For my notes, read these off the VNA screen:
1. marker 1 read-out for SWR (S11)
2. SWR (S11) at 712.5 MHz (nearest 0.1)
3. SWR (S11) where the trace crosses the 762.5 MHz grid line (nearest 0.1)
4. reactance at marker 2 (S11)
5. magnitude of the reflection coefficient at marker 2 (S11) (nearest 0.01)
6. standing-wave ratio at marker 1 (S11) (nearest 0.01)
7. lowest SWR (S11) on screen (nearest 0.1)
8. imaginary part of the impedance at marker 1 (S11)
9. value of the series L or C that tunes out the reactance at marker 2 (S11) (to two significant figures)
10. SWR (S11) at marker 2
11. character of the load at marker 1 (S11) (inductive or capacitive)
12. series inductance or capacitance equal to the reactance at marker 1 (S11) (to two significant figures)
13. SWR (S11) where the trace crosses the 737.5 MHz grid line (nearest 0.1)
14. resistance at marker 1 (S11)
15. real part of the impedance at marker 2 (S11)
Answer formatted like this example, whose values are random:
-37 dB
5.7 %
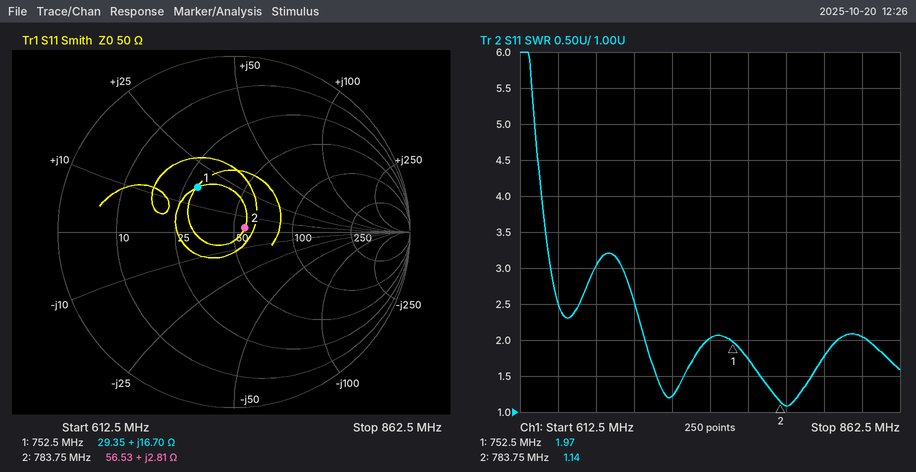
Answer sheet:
1.97
1.2
1.7
+2.81 Ω
0.07
1.97
1.1
+16.70 Ω
72 pF
1.14
inductive
3.5 nH
2.0
29.35 Ω
56.53 Ω
